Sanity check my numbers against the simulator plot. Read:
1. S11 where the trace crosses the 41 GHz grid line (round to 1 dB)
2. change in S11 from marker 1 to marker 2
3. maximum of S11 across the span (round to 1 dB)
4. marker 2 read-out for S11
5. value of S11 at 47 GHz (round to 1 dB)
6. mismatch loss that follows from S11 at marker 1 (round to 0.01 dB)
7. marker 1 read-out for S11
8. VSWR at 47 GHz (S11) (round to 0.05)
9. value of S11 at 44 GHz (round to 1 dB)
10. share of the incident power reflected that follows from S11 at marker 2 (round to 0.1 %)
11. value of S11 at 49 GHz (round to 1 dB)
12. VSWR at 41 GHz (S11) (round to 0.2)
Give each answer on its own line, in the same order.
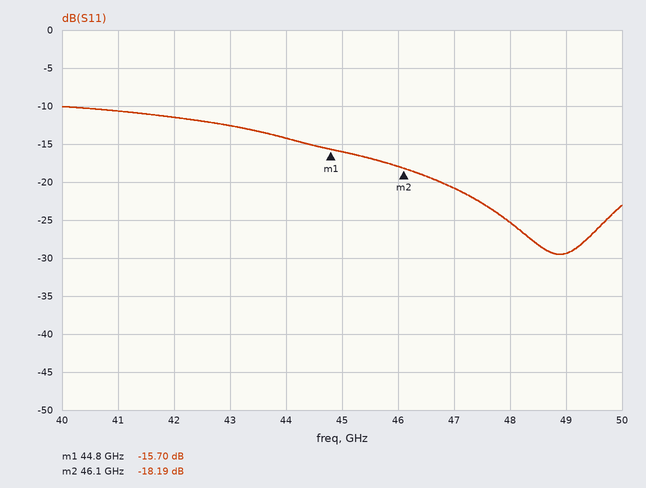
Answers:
-11 dB
-2.49 dB
-10 dB
-18.19 dB
-21 dB
0.12 dB
-15.70 dB
1.20
-14 dB
1.5 %
-29 dB
1.8
